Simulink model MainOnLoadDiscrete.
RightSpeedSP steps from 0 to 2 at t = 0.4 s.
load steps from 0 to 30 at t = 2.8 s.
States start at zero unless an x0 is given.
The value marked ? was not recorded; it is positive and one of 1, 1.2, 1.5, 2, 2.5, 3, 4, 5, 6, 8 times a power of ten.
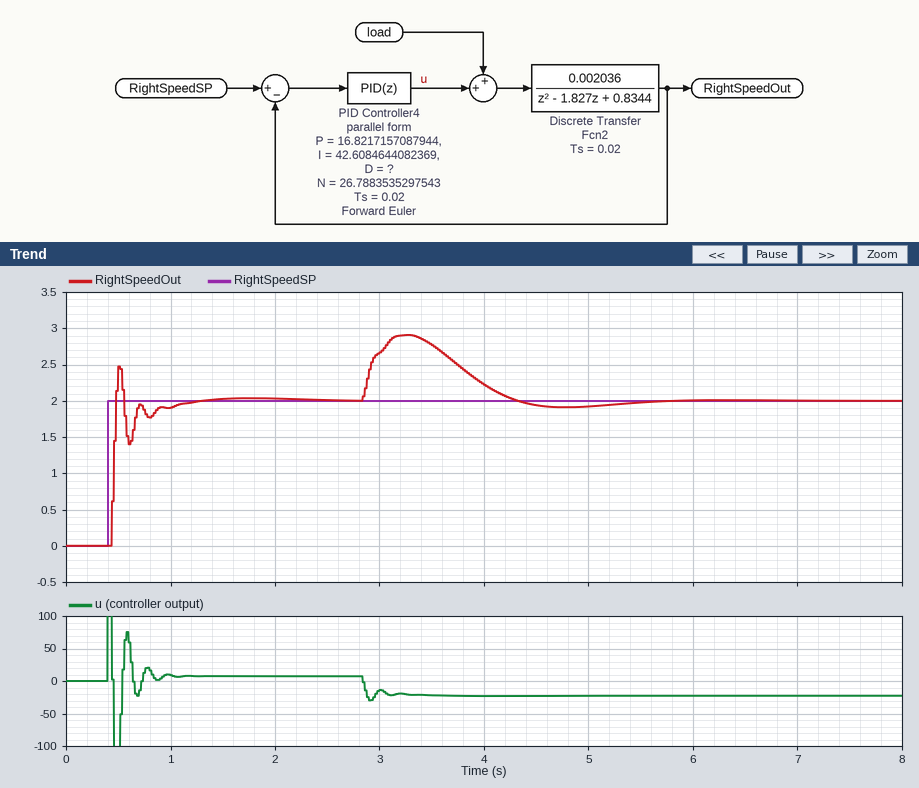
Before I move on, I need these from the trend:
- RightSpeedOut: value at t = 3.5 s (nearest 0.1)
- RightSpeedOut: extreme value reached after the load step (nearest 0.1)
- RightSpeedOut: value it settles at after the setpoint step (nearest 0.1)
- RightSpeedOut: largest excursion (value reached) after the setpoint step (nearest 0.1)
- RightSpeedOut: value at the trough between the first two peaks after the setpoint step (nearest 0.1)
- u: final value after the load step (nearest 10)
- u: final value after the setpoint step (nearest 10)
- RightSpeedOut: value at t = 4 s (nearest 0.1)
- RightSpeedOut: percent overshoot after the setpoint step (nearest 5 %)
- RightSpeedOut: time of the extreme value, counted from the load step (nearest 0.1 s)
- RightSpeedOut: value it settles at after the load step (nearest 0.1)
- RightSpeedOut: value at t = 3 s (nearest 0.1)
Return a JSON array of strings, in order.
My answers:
["2.8", "2.9", "2.0", "2.5", "1.4", "-20", "10", "2.2", "25 %", "0.5 s", "2.0", "2.7"]
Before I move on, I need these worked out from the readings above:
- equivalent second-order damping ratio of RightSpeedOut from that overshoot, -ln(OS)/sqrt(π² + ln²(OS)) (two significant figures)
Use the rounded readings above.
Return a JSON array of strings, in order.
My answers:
["0.40"]
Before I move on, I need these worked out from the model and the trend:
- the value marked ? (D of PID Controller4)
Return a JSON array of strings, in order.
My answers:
["5"]
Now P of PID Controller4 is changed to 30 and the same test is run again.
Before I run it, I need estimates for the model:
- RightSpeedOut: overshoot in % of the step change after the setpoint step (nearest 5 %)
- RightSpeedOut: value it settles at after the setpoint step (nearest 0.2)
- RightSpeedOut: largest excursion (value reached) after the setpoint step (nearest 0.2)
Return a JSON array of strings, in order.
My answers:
["40 %", "2.0", "2.8"]
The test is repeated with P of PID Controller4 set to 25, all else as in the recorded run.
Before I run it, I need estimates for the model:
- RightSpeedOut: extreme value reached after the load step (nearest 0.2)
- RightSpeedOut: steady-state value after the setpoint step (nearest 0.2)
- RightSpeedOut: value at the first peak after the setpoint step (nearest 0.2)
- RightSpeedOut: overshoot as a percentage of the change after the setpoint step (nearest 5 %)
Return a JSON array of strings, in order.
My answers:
["2.8", "2.0", "2.6", "35 %"]
